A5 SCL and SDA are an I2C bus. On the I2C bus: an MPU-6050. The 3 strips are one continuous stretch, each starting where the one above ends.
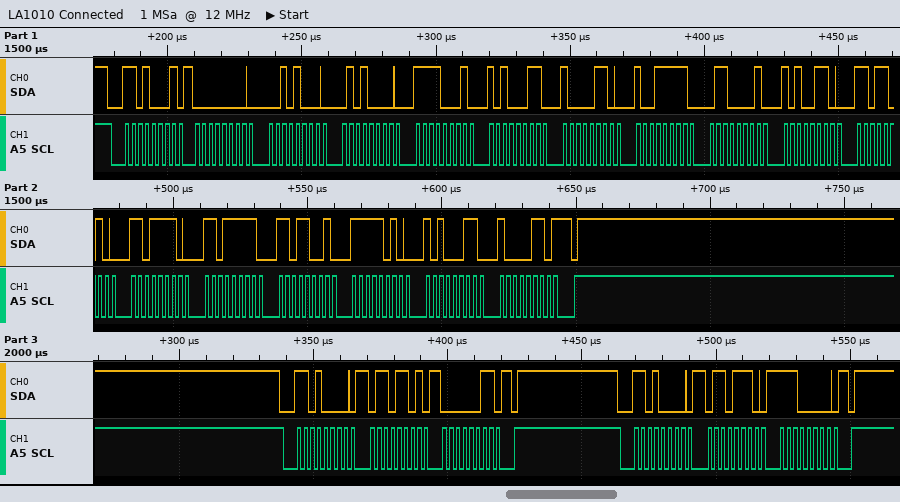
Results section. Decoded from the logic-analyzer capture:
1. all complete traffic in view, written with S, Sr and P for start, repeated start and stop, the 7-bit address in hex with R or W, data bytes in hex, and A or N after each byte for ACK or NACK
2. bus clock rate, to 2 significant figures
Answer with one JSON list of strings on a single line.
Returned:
["S 68R A 00 A 28 A 50 A F1 A A3 A 86 A 9F A 61 A A6 A DA A DE A DF A D9 A FA A A3 A 86 N P S 68W A 6D A 03 A P S 68W A 6E A E0 A P", "400 kHz"]
